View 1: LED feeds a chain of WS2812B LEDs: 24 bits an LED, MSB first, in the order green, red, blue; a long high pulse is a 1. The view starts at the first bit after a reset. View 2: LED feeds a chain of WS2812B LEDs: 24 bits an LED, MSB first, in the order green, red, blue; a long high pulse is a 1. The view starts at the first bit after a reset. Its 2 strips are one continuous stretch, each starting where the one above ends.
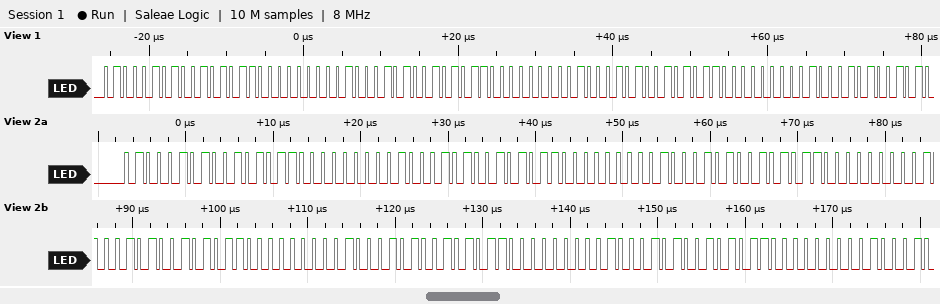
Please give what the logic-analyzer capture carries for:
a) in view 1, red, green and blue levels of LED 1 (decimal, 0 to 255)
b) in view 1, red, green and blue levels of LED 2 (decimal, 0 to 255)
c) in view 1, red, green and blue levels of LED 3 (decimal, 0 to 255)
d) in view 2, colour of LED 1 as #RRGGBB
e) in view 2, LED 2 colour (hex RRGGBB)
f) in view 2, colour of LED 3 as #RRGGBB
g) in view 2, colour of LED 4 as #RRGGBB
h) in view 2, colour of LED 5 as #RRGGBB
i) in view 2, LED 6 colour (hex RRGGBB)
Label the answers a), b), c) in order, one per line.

a) 43, 69, 0
b) 43, 69, 0
c) 43, 69, 0
d) #2B4500
e) #2B4500
f) #2B4500
g) #2B4500
h) #2B4500
i) #2B4500
